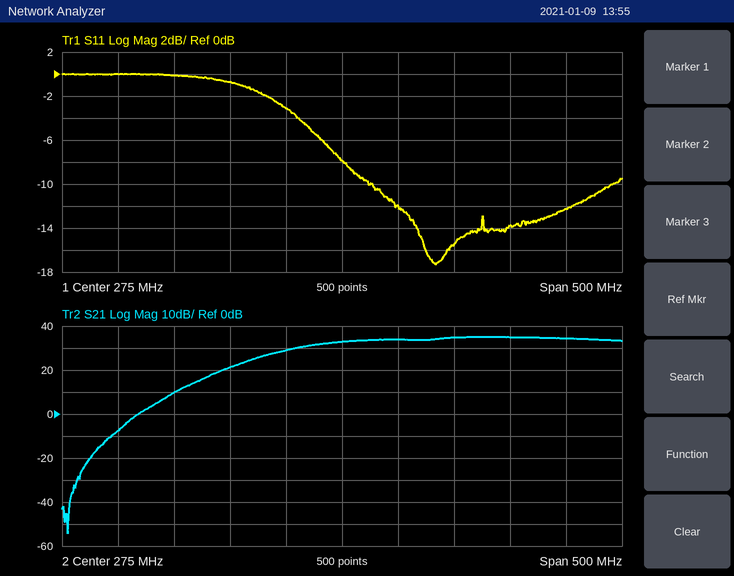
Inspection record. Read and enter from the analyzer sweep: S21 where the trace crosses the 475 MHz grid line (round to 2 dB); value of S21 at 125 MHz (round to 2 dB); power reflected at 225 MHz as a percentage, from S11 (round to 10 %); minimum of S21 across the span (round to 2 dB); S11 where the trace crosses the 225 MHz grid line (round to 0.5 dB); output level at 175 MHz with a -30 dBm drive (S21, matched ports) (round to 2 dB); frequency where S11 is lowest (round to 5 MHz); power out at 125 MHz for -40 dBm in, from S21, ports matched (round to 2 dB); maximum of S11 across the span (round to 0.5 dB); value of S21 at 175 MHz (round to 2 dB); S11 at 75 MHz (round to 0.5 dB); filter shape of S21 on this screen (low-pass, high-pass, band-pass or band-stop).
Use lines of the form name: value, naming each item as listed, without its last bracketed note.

S21 where the trace crosses the 475 MHz grid line: 34 dB
value of S21 at 125 MHz: 10 dB
power reflected at 225 MHz as a percentage, from S11: 50 %
minimum of S21 across the span: -54 dB
S11 where the trace crosses the 225 MHz grid line: -3.0 dB
output level at 175 MHz with a -30 dBm drive (S21, matched ports): -8 dBm
frequency where S11 is lowest: 360 MHz
power out at 125 MHz for -40 dBm in, from S21, ports matched: -30 dBm
maximum of S11 across the span: 0.0 dB
value of S21 at 175 MHz: 22 dB
S11 at 75 MHz: 0.0 dB
filter shape of S21 on this screen: high-pass
